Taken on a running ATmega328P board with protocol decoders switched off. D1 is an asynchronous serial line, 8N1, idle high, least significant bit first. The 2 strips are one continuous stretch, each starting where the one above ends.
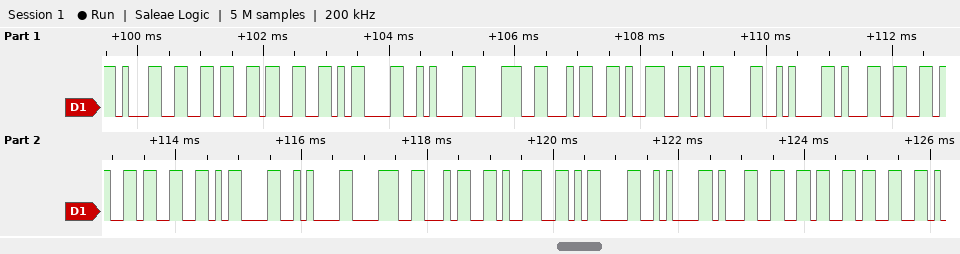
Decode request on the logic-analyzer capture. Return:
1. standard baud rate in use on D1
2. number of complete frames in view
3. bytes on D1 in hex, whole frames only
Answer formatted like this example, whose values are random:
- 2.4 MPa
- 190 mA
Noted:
- 9600 baud
- 23
- 0x31 0x36 0x33 0x0D 0x0A 0x38 0x34 0x39 0x0D 0x0A 0x31 0x36 0x33 0x0D 0x0A 0x38 0x34 0x39 0x0D 0x0A 0x31 0x36 0x33
